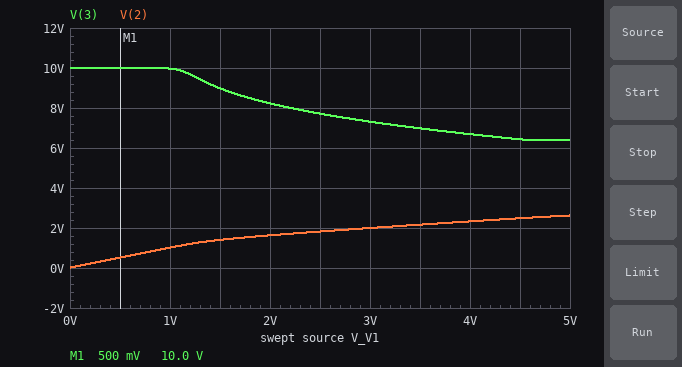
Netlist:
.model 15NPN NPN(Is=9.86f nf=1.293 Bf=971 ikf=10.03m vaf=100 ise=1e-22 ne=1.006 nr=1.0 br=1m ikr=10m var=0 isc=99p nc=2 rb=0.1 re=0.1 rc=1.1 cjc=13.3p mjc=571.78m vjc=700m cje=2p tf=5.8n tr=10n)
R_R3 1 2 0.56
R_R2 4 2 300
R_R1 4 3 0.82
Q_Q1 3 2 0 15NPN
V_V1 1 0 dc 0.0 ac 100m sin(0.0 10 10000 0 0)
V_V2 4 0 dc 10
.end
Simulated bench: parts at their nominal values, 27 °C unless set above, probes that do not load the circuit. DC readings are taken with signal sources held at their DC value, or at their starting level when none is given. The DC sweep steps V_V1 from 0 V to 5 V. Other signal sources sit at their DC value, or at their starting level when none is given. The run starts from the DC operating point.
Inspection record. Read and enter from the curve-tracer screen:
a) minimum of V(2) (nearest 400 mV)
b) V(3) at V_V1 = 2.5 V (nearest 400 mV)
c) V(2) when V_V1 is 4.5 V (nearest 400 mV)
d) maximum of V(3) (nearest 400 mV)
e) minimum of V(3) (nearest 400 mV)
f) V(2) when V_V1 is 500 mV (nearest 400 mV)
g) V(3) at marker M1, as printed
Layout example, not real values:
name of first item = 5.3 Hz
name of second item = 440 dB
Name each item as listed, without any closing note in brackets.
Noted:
minimum of V(2) = 0 V
V(3) at V_V1 = 2.5 V = 7.6 V
V(2) when V_V1 is 4.5 V = 2.4 V
maximum of V(3) = 10.0 V
minimum of V(3) = 6.4 V
V(2) when V_V1 is 500 mV = 400 mV
V(3) at marker M1, as printed = 10.0 V
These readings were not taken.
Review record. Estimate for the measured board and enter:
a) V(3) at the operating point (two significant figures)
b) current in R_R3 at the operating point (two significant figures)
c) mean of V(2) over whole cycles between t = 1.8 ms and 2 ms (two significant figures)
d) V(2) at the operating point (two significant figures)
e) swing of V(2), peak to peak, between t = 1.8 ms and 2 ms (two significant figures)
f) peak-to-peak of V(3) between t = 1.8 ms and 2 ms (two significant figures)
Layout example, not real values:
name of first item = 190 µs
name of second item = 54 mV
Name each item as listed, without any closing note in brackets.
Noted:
V(3) at the operating point = 10 V
current in R_R3 at the operating point = 33 mA
mean of V(2) over whole cycles between t = 1.8 ms and 2 ms = -1.7 V
V(2) at the operating point = 19 mV
swing of V(2), peak to peak, between t = 1.8 ms and 2 ms = 14 V
peak-to-peak of V(3) between t = 1.8 ms and 2 ms = 3.6 V
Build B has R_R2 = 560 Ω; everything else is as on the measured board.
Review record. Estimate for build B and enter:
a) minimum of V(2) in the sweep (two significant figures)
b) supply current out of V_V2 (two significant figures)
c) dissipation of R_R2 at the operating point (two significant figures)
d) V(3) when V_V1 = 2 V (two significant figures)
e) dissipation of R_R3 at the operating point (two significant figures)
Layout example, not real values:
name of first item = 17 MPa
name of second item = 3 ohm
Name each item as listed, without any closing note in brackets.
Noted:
minimum of V(2) in the sweep = 10 mV
supply current out of V_V2 = 18 mA
dissipation of R_R2 at the operating point = 180 mW
V(3) when V_V1 = 2 V = 8.2 V
dissipation of R_R3 at the operating point = 180 µW
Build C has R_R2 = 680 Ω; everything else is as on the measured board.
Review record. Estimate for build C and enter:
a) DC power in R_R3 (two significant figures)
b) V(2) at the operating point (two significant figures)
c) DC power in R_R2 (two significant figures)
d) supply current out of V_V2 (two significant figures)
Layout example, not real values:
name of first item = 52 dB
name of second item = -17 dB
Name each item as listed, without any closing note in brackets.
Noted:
DC power in R_R3 = 120 µW
V(2) at the operating point = 8.2 mV
DC power in R_R2 = 150 mW
supply current out of V_V2 = 15 mA
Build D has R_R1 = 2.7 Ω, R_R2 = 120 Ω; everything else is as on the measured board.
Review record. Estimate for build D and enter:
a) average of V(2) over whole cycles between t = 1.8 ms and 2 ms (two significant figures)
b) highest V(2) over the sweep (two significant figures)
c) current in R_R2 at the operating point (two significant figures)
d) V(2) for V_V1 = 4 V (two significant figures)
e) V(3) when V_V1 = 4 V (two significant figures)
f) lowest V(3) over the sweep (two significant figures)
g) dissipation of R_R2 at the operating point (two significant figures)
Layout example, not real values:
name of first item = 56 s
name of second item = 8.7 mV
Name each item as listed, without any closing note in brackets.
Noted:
average of V(2) over whole cycles between t = 1.8 ms and 2 ms = -1.8 V
highest V(2) over the sweep = 2.5 V
current in R_R2 at the operating point = 83 mA
V(2) for V_V1 = 4 V = 2.2 V
V(3) when V_V1 = 4 V = 3.8 V
lowest V(3) over the sweep = 3.6 V
dissipation of R_R2 at the operating point = 830 mW
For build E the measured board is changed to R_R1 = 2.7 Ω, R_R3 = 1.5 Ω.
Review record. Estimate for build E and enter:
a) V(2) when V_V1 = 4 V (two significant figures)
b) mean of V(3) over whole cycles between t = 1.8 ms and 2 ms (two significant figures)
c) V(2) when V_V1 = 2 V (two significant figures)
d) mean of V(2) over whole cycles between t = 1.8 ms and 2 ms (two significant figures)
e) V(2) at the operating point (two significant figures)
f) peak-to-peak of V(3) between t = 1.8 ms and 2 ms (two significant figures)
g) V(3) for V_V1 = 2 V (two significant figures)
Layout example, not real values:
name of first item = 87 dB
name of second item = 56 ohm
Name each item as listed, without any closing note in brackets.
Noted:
V(2) when V_V1 = 4 V = 1.8 V
mean of V(3) over whole cycles between t = 1.8 ms and 2 ms = 7.2 V
V(2) when V_V1 = 2 V = 1.5 V
mean of V(2) over whole cycles between t = 1.8 ms and 2 ms = -2.1 V
V(2) at the operating point = 50 mV
peak-to-peak of V(3) between t = 1.8 ms and 2 ms = 6.4 V
V(3) for V_V1 = 2 V = 5.7 V
